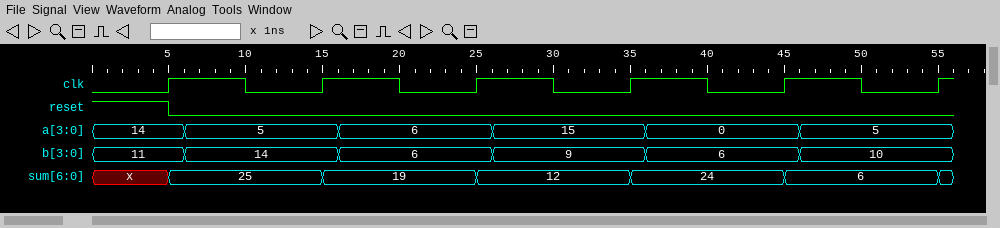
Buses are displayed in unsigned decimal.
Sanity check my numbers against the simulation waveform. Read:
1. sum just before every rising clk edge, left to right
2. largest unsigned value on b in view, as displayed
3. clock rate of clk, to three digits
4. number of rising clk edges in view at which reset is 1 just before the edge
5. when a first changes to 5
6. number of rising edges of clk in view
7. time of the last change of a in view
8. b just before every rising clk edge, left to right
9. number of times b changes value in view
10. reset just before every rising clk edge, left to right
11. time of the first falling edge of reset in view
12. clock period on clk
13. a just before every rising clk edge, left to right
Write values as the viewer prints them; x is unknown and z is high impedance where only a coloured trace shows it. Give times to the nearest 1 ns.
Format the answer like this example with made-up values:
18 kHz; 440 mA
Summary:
x, 25, 19, 12, 24, 6; 14; 100 MHz; 1; 6 ns; 6; 46 ns; 11, 14, 6, 9, 6, 10; 5; 1 0 0 0 0 0; 5 ns; 10 ns; 14, 5, 6, 15, 0, 5
